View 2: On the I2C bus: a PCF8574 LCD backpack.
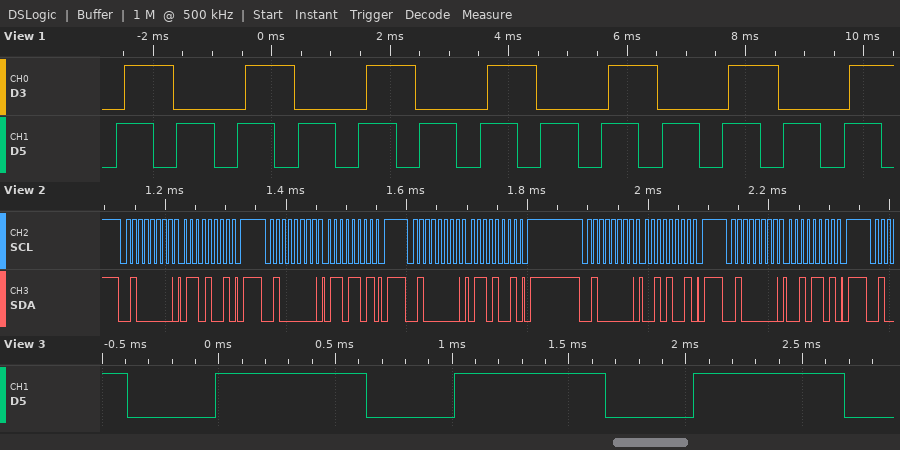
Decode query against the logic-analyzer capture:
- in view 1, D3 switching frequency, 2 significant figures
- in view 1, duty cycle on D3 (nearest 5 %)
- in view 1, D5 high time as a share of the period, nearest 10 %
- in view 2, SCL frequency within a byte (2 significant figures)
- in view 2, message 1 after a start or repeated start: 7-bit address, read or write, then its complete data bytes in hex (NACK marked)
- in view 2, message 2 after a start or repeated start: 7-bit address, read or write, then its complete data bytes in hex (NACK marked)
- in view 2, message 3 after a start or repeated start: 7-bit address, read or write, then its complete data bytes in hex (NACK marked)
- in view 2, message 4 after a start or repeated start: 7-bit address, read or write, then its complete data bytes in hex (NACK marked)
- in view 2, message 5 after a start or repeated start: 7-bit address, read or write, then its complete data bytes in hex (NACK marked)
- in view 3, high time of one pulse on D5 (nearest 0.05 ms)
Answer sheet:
490 Hz
40 %
60 %
100 kHz
0x20 write: 69
0x20 write: 6D
0x20 write: 69
0x20 write: 29
0x20 write: 2D
0.65 ms
